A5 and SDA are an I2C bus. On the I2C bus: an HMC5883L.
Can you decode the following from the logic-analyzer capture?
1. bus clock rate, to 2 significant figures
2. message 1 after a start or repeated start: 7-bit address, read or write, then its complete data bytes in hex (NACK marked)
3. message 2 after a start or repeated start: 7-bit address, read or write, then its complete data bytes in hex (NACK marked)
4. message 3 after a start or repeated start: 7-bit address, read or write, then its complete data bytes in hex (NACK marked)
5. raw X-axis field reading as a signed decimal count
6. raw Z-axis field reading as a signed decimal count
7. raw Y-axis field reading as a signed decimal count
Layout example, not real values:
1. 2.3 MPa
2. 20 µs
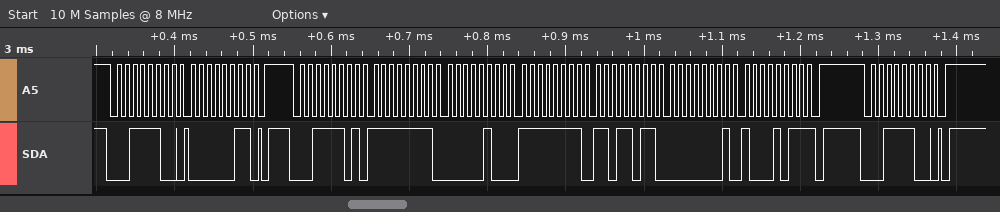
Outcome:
1. 100 kHz
2. 0x1E write: 03
3. 0x1E read: FF 04 FF DB 01 8B NACK
4. 0x1E write
5. -252
6. -37
7. 395
